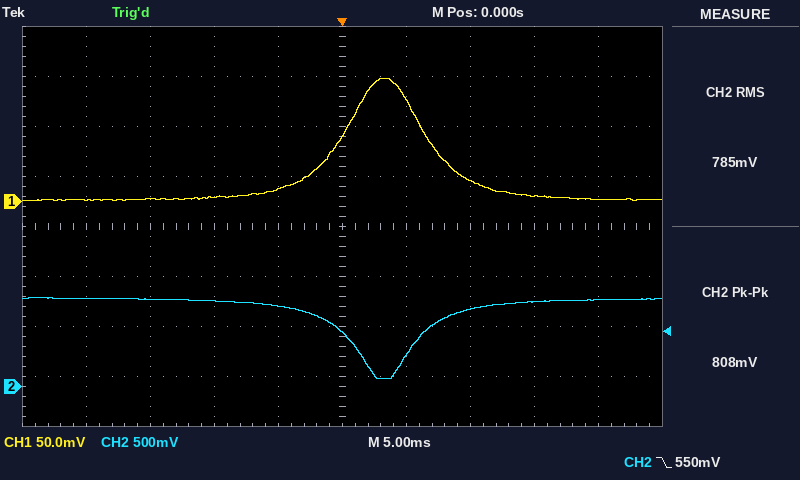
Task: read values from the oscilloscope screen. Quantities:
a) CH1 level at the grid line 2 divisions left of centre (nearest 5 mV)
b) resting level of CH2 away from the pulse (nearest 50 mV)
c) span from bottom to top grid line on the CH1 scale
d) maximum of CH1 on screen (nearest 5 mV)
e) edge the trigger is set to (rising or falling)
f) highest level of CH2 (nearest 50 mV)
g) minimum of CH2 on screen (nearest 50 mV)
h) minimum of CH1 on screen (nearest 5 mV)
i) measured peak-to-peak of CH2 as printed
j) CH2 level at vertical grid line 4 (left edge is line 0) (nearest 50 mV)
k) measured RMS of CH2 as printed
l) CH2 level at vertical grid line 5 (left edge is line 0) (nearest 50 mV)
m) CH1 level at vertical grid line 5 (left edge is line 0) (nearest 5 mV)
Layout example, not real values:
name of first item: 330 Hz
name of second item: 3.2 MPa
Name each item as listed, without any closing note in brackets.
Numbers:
CH1 level at the grid line 2 divisions left of centre: 5 mV
resting level of CH2 away from the pulse: 850 mV
span from bottom to top grid line on the CH1 scale: 400 mV
maximum of CH1 on screen: 125 mV
edge the trigger is set to: falling
highest level of CH2: 900 mV
minimum of CH2 on screen: 100 mV
minimum of CH1 on screen: 0 mV
measured peak-to-peak of CH2 as printed: 808 mV
CH2 level at vertical grid line 4 (left edge is line 0): 800 mV
measured RMS of CH2 as printed: 785 mV
CH2 level at vertical grid line 5 (left edge is line 0): 550 mV
CH1 level at vertical grid line 5 (left edge is line 0): 65 mV
